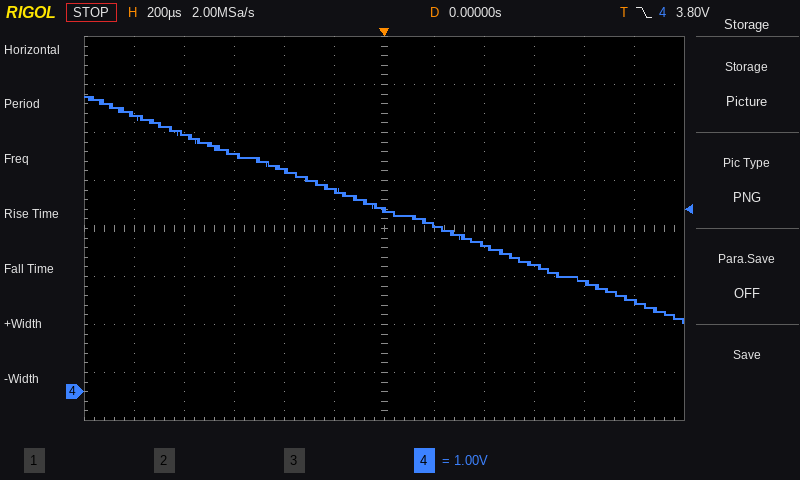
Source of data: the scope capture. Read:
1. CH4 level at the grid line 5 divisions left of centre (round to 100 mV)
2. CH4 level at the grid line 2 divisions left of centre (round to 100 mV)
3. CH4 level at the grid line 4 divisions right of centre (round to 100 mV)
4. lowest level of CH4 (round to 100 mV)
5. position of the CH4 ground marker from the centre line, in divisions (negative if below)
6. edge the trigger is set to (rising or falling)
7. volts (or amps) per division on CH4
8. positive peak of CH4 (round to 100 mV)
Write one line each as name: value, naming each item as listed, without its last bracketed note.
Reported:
CH4 level at the grid line 5 divisions left of centre: 5.8 V
CH4 level at the grid line 2 divisions left of centre: 4.6 V
CH4 level at the grid line 4 divisions right of centre: 2.3 V
lowest level of CH4: 1.4 V
position of the CH4 ground marker from the centre line, in divisions: -3.4 div
edge the trigger is set to: falling
volts (or amps) per division on CH4: 1 V
positive peak of CH4: 6.2 V
